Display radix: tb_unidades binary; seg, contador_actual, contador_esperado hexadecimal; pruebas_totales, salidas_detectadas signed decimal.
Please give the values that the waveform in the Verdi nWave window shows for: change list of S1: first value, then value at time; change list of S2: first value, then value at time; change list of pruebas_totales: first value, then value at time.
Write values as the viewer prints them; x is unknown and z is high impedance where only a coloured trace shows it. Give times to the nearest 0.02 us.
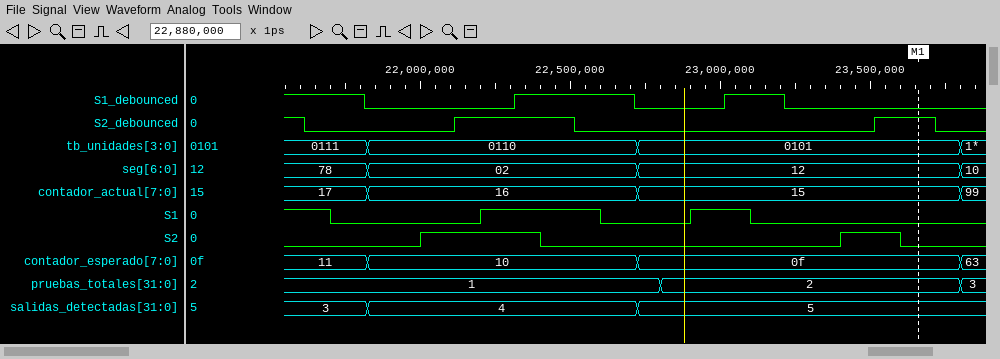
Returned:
1, 0 at 21.7 us, 1 at 22.2 us, 0 at 22.6 us, 1 at 22.9 us, 0 at 23.1 us
0, 1 at 22 us, 0 at 22.4 us, 1 at 23.4 us, 0 at 23.6 us
1, 2 at 22.8 us, 3 at 23.8 us
